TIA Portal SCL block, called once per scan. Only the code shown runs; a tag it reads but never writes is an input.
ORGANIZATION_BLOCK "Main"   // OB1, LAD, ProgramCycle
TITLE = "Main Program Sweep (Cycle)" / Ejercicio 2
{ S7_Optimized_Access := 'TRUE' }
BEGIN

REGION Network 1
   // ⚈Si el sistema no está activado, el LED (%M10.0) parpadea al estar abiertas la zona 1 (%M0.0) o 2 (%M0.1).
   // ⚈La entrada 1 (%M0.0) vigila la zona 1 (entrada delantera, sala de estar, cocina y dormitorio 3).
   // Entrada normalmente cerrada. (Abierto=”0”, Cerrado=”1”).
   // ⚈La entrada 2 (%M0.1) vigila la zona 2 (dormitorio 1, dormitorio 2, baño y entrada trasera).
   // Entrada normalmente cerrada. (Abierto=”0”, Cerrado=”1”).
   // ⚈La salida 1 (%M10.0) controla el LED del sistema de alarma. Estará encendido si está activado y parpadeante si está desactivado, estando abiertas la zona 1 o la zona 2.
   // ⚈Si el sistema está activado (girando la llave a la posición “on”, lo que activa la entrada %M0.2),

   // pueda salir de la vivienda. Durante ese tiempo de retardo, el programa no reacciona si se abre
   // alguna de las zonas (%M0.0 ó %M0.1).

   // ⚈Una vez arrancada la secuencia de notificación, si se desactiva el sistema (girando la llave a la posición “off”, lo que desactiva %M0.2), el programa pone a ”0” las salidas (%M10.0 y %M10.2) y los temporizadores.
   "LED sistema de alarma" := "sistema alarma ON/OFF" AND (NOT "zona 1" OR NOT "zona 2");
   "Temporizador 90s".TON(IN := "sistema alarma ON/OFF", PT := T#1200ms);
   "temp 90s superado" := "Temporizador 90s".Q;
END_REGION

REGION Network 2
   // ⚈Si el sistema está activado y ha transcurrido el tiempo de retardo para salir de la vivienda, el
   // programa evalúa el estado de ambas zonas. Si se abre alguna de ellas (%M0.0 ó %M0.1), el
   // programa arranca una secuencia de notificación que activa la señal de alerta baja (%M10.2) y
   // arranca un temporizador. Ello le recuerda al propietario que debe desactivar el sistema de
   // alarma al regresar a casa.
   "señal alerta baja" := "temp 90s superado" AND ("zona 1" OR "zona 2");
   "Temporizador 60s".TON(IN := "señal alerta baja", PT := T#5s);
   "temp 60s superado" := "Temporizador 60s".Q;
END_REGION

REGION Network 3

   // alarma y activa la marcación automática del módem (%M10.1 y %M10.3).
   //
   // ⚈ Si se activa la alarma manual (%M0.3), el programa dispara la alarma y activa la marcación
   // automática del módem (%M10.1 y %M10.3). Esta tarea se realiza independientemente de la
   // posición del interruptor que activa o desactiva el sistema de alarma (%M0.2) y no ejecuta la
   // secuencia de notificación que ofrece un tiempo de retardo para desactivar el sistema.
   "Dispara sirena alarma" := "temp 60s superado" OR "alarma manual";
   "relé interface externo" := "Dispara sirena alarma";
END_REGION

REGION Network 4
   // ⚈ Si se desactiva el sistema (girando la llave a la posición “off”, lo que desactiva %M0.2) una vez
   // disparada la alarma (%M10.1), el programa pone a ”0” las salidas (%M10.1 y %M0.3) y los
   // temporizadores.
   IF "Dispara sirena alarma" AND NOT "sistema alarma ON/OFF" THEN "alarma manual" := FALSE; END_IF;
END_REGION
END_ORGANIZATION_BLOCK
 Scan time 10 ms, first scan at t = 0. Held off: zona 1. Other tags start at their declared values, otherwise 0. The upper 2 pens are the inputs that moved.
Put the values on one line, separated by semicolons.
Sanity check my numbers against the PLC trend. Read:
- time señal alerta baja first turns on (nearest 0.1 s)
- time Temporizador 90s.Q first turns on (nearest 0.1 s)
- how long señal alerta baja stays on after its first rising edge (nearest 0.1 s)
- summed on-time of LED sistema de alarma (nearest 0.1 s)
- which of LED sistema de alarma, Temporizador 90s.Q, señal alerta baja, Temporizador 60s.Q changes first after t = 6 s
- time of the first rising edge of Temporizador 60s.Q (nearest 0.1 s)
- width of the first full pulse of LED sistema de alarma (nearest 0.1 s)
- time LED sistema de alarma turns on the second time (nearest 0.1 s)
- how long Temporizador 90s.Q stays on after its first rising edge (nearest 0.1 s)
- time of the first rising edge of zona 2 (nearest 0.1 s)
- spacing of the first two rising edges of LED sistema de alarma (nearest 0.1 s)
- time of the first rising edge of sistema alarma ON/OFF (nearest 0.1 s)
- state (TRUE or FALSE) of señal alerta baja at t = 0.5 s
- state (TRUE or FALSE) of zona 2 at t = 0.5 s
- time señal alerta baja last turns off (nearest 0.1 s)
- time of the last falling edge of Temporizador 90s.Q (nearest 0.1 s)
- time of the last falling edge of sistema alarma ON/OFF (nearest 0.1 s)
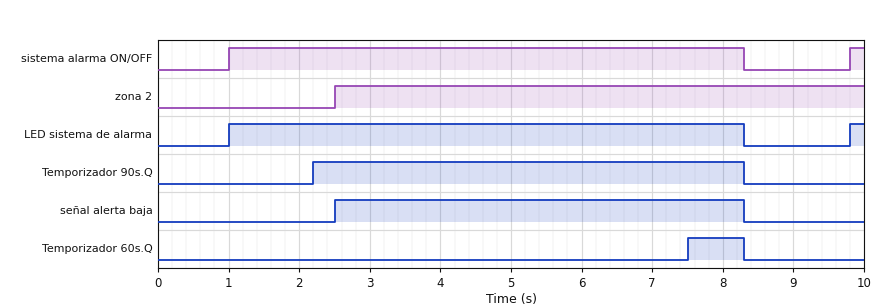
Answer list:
2.5 s; 2.2 s; 5.8 s; 7.5 s; Temporizador 60s.Q; 7.5 s; 7.3 s; 9.8 s; 6.1 s; 2.5 s; 8.8 s; 1.0 s; FALSE; FALSE; 8.3 s; 8.3 s; 8.3 s
